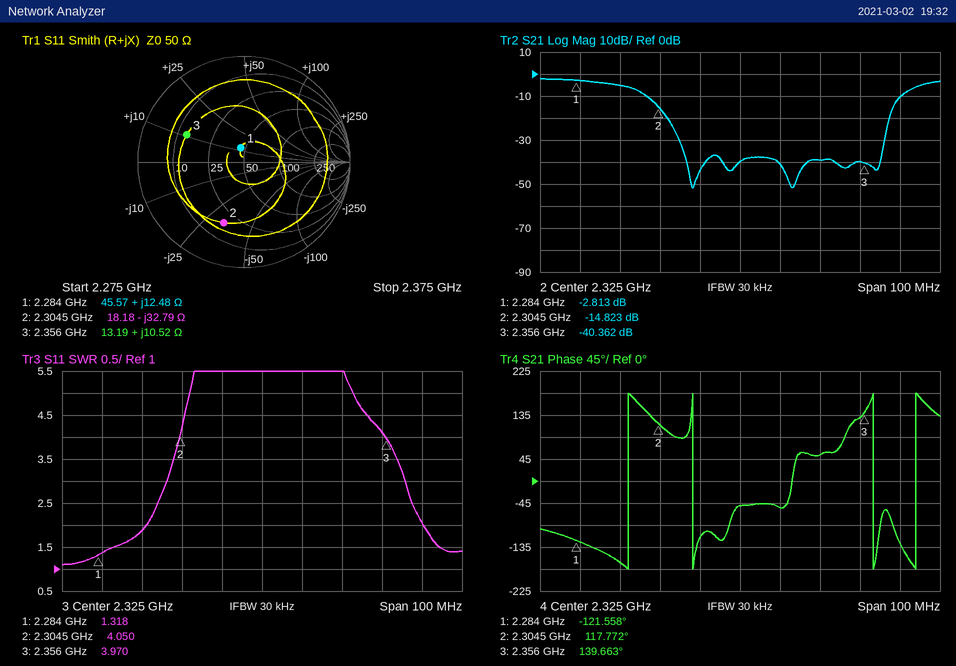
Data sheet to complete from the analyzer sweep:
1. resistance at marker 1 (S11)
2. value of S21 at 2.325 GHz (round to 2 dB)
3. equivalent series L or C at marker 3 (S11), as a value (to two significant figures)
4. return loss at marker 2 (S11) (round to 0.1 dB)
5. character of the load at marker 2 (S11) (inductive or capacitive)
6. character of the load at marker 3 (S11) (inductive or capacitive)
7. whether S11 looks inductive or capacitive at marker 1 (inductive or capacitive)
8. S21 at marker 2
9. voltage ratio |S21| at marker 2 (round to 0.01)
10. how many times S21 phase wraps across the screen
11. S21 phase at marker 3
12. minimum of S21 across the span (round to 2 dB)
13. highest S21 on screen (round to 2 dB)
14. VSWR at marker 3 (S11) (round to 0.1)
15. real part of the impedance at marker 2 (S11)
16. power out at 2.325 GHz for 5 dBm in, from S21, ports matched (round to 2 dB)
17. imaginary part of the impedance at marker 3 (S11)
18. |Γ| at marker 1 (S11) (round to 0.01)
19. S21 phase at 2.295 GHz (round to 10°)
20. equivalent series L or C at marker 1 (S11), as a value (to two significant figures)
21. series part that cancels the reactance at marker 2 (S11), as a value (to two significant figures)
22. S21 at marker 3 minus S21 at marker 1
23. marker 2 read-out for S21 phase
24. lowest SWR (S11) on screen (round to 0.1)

45.57 Ω
-40 dB
710 pH
4.4 dB
capacitive
inductive
inductive
-14.823 dB
0.18
4
139.663°
-52 dB
-2 dB
4.0
18.18 Ω
-34 dBm
+10.52 Ω
0.14
-170°
870 pH
2.3 nH
-37.549 dB
117.772°
1.1
